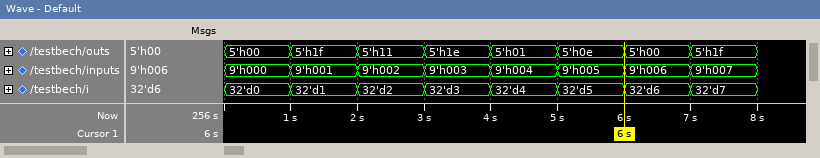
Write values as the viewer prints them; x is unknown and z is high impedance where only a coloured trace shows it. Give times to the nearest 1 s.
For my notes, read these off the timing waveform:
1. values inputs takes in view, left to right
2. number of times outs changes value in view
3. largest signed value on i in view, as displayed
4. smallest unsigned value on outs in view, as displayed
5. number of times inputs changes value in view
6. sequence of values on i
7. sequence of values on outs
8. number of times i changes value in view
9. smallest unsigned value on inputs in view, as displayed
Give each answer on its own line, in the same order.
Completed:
9'h000, 9'h001, 9'h002, 9'h003, 9'h004, 9'h005, 9'h006, 9'h007
7
32'd7
5'h00
7
32'd0, 32'd1, 32'd2, 32'd3, 32'd4, 32'd5, 32'd6, 32'd7
5'h00, 5'h1f, 5'h11, 5'h1e, 5'h01, 5'h0e, 5'h00, 5'h1f
7
9'h000
